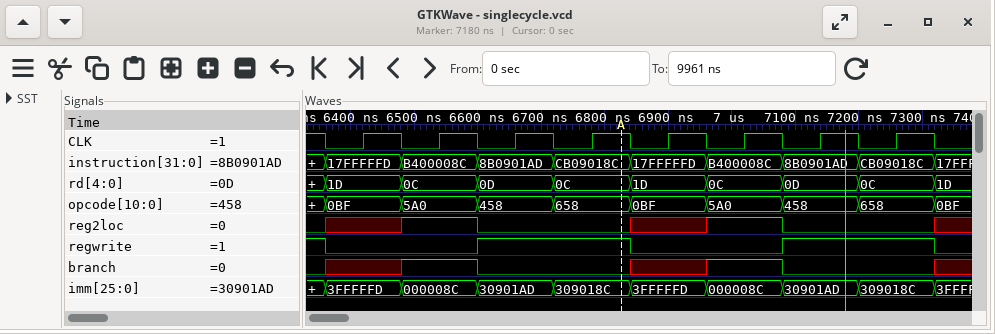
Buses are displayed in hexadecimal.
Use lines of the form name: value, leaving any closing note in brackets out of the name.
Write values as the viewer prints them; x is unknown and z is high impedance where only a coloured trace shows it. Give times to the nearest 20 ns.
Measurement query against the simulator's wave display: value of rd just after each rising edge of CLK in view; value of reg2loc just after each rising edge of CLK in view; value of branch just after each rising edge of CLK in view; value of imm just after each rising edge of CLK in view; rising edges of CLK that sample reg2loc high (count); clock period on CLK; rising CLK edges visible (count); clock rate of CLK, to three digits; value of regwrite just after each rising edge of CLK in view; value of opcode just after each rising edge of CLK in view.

value of rd just after each rising edge of CLK in view: 1D, 0C, 0D, 0C, 1D, 0C, 0D, 0C
value of reg2loc just after each rising edge of CLK in view: x 1 0 0 x 1 0 0
value of branch just after each rising edge of CLK in view: x 1 0 0 x 1 0 0
value of imm just after each rising edge of CLK in view: 3FFFFFD, 000008C, 30901AD, 309018C, 3FFFFFD, 000008C, 30901AD, 309018C
rising edges of CLK that sample reg2loc high: 2
clock period on CLK: 120 ns
rising CLK edges visible: 8
clock rate of CLK, to three digits: 8.33 MHz
value of regwrite just after each rising edge of CLK in view: 0 0 1 1 0 0 1 1
value of opcode just after each rising edge of CLK in view: 0BF, 5A0, 458, 658, 0BF, 5A0, 458, 658
